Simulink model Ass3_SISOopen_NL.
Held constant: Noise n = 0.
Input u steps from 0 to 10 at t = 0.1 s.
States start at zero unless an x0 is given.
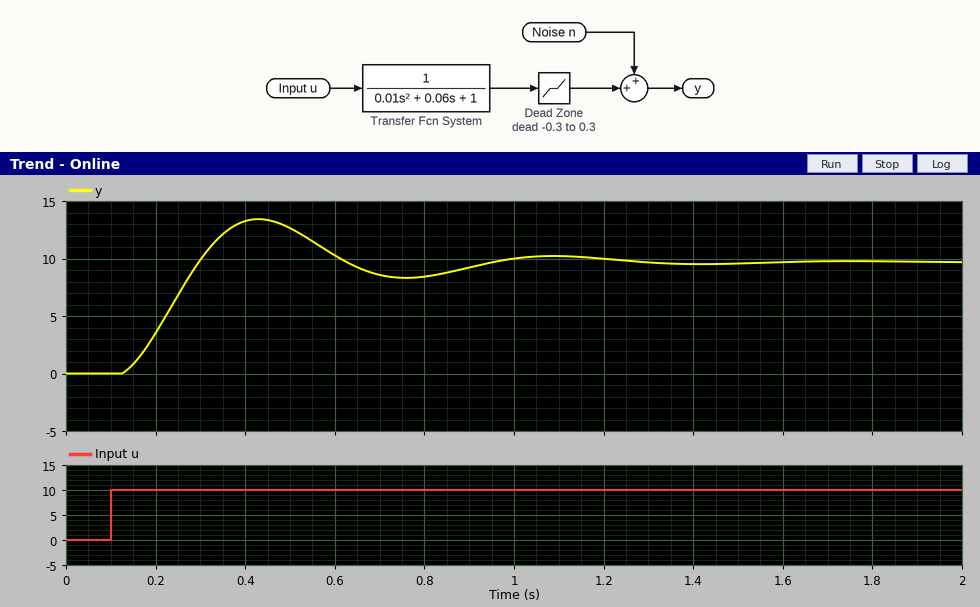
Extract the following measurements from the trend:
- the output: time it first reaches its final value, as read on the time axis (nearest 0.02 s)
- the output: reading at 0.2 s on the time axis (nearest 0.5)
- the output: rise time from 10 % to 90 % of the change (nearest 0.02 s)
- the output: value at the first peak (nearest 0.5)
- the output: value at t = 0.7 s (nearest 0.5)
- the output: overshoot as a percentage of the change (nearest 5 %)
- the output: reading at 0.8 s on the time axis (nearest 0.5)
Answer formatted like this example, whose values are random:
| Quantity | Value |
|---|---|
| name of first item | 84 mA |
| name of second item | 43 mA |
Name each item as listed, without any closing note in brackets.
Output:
| Quantity | Value |
|---|---|
| the output: time it first reaches its final value, as read on the time axis | 0.30 s |
| the output: reading at 0.2 s on the time axis | 3.5 |
| the output: rise time from 10 % to 90 % of the change | 0.12 s |
| the output: value at the first peak | 13.5 |
| the output: value at t = 0.7 s | 8.5 |
| the output: overshoot as a percentage of the change | 40 % |
| the output: reading at 0.8 s on the time axis | 8.5 |
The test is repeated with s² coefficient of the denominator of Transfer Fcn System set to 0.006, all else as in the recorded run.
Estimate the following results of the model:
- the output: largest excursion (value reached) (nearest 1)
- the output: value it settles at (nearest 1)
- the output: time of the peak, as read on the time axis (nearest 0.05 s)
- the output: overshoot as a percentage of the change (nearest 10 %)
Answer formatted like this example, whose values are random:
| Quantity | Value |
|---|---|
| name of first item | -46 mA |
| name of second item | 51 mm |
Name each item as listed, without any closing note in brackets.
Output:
| Quantity | Value |
|---|---|
| the output: largest excursion (value reached) | 12 |
| the output: value it settles at | 10 |
| the output: time of the peak, as read on the time axis | 0.35 s |
| the output: overshoot as a percentage of the change | 30 % |
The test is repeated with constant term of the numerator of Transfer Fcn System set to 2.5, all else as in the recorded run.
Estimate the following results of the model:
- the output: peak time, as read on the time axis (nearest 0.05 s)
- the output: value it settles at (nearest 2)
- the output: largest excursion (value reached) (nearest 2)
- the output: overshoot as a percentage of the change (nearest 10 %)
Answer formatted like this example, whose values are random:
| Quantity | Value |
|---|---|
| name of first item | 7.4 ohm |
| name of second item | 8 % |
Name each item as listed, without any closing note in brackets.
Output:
| Quantity | Value |
|---|---|
| the output: peak time, as read on the time axis | 0.45 s |
| the output: value it settles at | 24 |
| the output: largest excursion (value reached) | 34 |
| the output: overshoot as a percentage of the change | 40 % |
